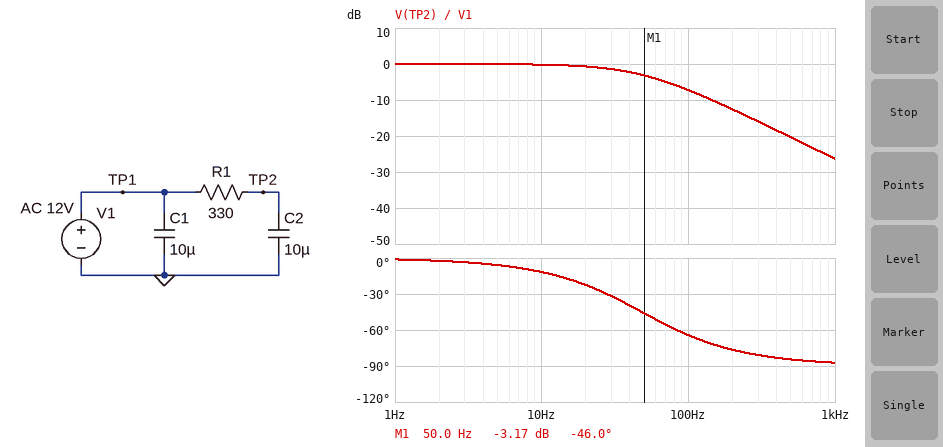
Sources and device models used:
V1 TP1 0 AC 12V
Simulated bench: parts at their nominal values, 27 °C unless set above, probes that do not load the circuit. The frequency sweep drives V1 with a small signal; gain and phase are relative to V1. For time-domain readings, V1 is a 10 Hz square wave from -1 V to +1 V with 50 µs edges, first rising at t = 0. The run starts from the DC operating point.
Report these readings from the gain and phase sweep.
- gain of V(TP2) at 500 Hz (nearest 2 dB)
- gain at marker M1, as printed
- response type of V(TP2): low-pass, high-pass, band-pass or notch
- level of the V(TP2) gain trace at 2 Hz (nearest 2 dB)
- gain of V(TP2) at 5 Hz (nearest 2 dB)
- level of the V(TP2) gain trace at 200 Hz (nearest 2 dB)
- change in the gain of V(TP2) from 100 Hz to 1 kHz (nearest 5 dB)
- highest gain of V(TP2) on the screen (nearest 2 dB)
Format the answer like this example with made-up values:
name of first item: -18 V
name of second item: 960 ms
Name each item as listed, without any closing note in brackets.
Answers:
gain of V(TP2) at 500 Hz: -20 dB
gain at marker M1, as printed: -3.17 dB
response type of V(TP2): low-pass, high-pass, band-pass or notch: low-pass
level of the V(TP2) gain trace at 2 Hz: 0 dB
gain of V(TP2) at 5 Hz: 0 dB
level of the V(TP2) gain trace at 200 Hz: -12 dB
change in the gain of V(TP2) from 100 Hz to 1 kHz: -20 dB
highest gain of V(TP2) on the screen: 0 dB
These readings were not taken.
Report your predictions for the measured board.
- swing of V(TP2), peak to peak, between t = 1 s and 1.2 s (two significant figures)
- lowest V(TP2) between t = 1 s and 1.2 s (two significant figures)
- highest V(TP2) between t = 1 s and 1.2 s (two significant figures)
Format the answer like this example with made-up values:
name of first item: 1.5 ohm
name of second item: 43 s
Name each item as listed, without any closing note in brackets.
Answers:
swing of V(TP2), peak to peak, between t = 1 s and 1.2 s: 2.0 V
lowest V(TP2) between t = 1 s and 1.2 s: -1.0 V
highest V(TP2) between t = 1 s and 1.2 s: 1.0 V
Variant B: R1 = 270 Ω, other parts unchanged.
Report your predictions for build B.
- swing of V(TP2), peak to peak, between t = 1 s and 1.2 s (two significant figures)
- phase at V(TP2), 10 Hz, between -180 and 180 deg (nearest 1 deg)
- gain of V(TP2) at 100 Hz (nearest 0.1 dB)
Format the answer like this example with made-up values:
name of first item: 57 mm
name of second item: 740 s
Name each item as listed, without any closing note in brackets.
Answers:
swing of V(TP2), peak to peak, between t = 1 s and 1.2 s: 2.0 V
phase at V(TP2), 10 Hz, between -180 and 180 deg: -10 deg
gain of V(TP2) at 100 Hz: -5.9 dB
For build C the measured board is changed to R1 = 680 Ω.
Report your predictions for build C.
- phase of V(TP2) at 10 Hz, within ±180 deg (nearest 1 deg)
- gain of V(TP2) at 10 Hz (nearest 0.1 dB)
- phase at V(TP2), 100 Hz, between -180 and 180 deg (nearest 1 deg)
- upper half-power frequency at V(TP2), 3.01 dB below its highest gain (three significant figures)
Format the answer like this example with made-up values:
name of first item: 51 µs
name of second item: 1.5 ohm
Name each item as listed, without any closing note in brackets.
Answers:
phase of V(TP2) at 10 Hz, within ±180 deg: -23 deg
gain of V(TP2) at 10 Hz: -0.7 dB
phase at V(TP2), 100 Hz, between -180 and 180 deg: -77 deg
upper half-power frequency at V(TP2), 3.01 dB below its highest gain: 23.4 Hz
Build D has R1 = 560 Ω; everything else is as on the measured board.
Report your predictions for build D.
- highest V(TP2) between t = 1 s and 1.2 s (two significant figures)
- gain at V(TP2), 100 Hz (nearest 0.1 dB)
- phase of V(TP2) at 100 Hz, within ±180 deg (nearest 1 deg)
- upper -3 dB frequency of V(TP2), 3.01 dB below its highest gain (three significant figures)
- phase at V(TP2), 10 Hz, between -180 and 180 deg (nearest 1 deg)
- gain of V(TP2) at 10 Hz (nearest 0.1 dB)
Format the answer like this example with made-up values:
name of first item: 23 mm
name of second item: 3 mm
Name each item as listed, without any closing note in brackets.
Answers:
highest V(TP2) between t = 1 s and 1.2 s: 1.0 V
gain at V(TP2), 100 Hz: -11.3 dB
phase of V(TP2) at 100 Hz, within ±180 deg: -74 deg
upper -3 dB frequency of V(TP2), 3.01 dB below its highest gain: 28.4 Hz
phase at V(TP2), 10 Hz, between -180 and 180 deg: -19 deg
gain of V(TP2) at 10 Hz: -0.5 dB
